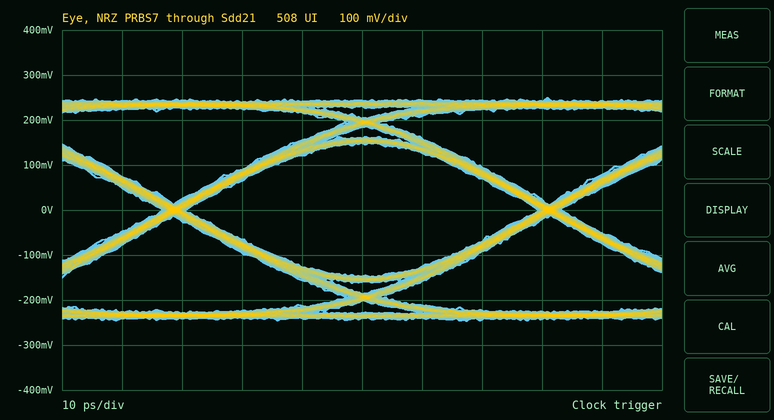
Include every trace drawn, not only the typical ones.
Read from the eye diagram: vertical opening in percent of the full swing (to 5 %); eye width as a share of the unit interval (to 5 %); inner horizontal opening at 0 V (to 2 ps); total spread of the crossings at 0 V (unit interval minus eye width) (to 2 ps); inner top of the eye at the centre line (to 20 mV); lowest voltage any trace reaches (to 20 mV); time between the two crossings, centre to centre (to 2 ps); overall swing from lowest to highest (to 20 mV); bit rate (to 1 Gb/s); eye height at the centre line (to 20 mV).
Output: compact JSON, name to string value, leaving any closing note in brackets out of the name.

{"vertical opening in percent of the full swing": "60 %", "eye width as a share of the unit interval": "95 %", "inner horizontal opening at 0 V": "58 ps", "total spread of the crossings at 0 V (unit interval minus eye width)": "4 ps", "inner top of the eye at the centre line": "140 mV", "lowest voltage any trace reaches": "-240 mV", "time between the two crossings, centre to centre": "62 ps", "overall swing from lowest to highest": "500 mV", "bit rate": "16 Gb/s", "eye height at the centre line": "300 mV"}
